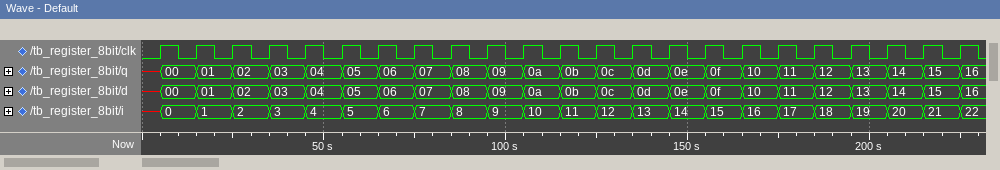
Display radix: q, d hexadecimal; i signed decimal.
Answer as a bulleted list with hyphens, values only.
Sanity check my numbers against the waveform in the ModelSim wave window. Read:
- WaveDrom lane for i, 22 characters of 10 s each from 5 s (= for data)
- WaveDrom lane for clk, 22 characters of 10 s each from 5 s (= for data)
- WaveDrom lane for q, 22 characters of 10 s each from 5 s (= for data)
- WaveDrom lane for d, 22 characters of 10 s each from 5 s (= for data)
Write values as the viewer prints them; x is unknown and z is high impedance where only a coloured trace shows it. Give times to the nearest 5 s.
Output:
- {name: 'i', wave: '======================', data: '0 1 2 3 4 5 6 7 8 9 10 11 12 13 14 15 16 17 18 19 20 21'}
- {name: 'clk', wave: 'p.....................'}
- {name: 'q', wave: '======================', data: '00 01 02 03 04 05 06 07 08 09 0a 0b 0c 0d 0e 0f 10 11 12 13 14 15'}
- {name: 'd', wave: '======================', data: '00 01 02 03 04 05 06 07 08 09 0a 0b 0c 0d 0e 0f 10 11 12 13 14 15'}
